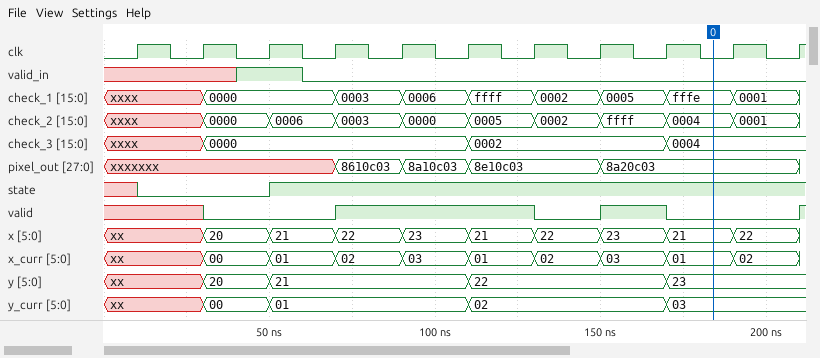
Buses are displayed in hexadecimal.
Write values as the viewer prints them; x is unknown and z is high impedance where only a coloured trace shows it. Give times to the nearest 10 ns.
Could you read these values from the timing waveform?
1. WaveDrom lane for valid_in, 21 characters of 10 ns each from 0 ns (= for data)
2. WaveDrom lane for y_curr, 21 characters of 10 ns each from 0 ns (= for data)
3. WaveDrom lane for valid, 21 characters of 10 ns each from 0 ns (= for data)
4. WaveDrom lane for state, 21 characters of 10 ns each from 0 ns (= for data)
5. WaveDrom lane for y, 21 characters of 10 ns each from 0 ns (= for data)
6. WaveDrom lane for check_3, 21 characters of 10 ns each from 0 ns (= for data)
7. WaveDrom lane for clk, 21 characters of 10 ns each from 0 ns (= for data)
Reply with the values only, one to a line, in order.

{name: 'valid_in', wave: 'x...1.0..............'}
{name: 'y_curr', wave: 'x..=.=.....=.....=...', data: '00 01 02 03'}
{name: 'valid', wave: 'x..0...1.....0.1.0...'}
{name: 'state', wave: 'x0...1...............'}
{name: 'y', wave: 'x..=.=.....=.....=...', data: '20 21 22 23'}
{name: 'check_3', wave: 'x..=.......=.....=...', data: '0000 0002 0004'}
{name: 'clk', wave: '010101010101010101010'}
